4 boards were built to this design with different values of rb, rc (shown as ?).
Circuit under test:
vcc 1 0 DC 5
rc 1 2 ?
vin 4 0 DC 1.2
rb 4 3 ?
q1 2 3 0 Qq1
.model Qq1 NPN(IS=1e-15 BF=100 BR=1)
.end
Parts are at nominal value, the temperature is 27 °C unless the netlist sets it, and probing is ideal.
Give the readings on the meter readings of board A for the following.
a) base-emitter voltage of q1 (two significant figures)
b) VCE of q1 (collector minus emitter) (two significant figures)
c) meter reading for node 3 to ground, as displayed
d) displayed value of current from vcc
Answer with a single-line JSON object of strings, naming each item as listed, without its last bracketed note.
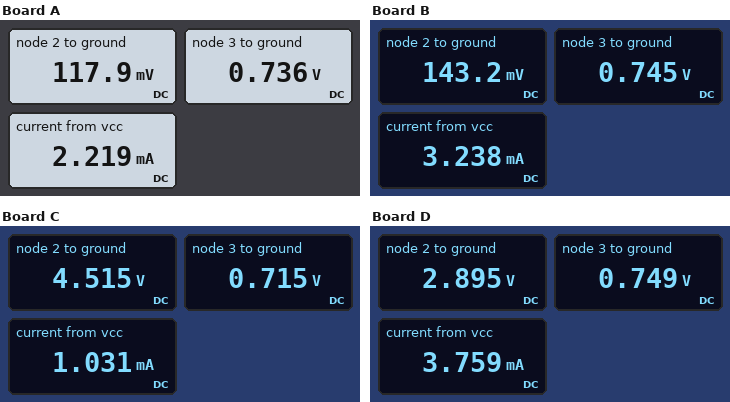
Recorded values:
{"base-emitter voltage of q1": "740 mV", "VCE of q1 (collector minus emitter)": "120 mV", "meter reading for node 3 to ground, as displayed": "0.736 V", "displayed value of current from vcc": "2.219 mA"}
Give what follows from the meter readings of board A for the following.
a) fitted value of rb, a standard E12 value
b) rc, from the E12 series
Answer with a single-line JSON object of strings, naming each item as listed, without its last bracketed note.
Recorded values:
{"fitted value of rb, a standard E12 value": "10 kΩ", "rc, from the E12 series": "2.2 kΩ"}
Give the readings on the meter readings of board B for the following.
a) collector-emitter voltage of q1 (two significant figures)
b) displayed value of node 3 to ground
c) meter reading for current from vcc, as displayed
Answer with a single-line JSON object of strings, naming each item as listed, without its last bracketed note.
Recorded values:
{"collector-emitter voltage of q1": "140 mV", "displayed value of node 3 to ground": "0.745 V", "meter reading for current from vcc, as displayed": "3.238 mA"}
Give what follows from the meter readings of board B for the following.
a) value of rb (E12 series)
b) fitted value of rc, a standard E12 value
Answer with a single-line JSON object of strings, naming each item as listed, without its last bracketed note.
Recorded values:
{"value of rb": "10 kΩ", "fitted value of rc, a standard E12 value": "1.5 kΩ"}
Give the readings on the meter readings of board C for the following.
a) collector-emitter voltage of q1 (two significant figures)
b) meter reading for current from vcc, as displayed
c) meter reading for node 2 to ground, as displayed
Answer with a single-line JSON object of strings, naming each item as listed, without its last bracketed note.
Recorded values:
{"collector-emitter voltage of q1": "4.5 V", "meter reading for current from vcc, as displayed": "1.031 mA", "meter reading for node 2 to ground, as displayed": "4.515 V"}
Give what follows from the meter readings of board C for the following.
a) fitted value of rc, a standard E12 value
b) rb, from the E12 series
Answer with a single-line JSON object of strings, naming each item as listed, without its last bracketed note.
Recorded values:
{"fitted value of rc, a standard E12 value": "470 Ω", "rb, from the E12 series": "47 kΩ"}
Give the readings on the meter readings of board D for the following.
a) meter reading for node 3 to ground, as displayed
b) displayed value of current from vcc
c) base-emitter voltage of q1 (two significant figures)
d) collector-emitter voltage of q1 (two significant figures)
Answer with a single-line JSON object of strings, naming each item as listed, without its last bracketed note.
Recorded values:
{"meter reading for node 3 to ground, as displayed": "0.749 V", "displayed value of current from vcc": "3.759 mA", "base-emitter voltage of q1": "750 mV", "collector-emitter voltage of q1": "2.9 V"}
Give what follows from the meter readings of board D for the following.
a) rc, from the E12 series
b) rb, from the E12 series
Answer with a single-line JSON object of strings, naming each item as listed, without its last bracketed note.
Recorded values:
{"rc, from the E12 series": "560 Ω", "rb, from the E12 series": "12 kΩ"}
